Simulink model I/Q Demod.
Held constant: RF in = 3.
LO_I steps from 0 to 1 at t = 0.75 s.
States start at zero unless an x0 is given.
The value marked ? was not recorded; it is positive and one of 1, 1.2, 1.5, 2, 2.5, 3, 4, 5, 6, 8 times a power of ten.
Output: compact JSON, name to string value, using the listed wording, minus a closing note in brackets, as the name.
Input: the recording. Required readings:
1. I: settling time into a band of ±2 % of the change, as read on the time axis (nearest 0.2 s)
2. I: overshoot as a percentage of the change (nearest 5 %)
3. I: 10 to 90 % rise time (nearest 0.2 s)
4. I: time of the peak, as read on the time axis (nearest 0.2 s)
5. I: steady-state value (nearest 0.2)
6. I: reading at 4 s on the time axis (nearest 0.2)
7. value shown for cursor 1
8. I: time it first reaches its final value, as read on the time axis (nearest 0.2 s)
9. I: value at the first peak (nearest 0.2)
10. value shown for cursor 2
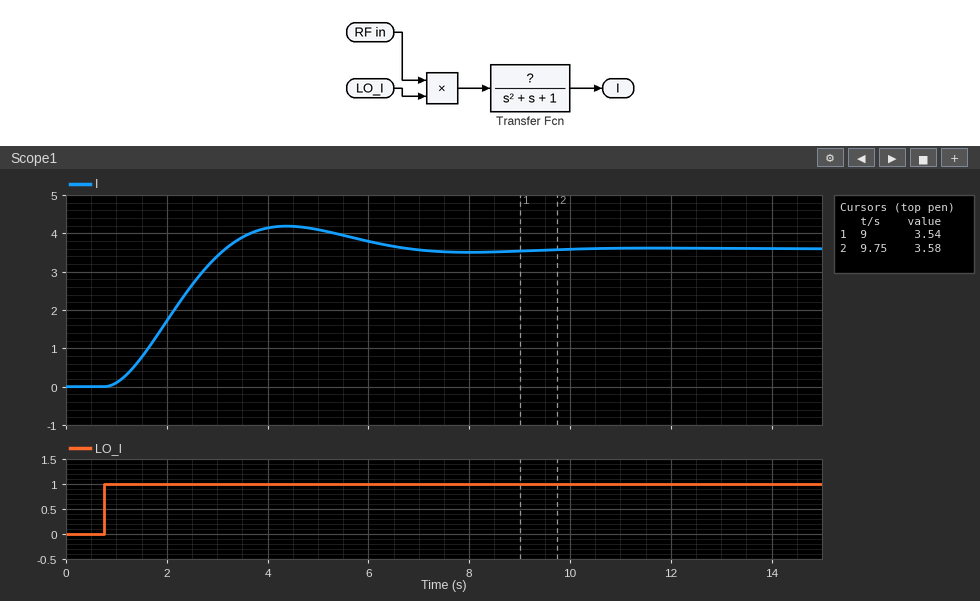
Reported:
{"I: settling time into a band of ±2 % of the change, as read on the time axis": "8.8 s", "I: overshoot as a percentage of the change": "15 %", "I: 10 to 90 % rise time": "1.6 s", "I: time of the peak, as read on the time axis": "4.4 s", "I: steady-state value": "3.6", "I: reading at 4 s on the time axis": "4.2", "value shown for cursor 1": "3.54", "I: time it first reaches its final value, as read on the time axis": "3.2 s", "I: value at the first peak": "4.2", "value shown for cursor 2": "3.58"}
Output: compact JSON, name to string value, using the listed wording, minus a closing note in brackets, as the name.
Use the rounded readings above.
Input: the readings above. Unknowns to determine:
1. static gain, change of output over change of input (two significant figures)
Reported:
{"static gain, change of output over change of input": "3.6"}
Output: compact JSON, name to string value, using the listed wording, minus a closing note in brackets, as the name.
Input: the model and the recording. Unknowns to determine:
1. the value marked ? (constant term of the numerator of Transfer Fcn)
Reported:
{"the value marked ?": "1.2"}
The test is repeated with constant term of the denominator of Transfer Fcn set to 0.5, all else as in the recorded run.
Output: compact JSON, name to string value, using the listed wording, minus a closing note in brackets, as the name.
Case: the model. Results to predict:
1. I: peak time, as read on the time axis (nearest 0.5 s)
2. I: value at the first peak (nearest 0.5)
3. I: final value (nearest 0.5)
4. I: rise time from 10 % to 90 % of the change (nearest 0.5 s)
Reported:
{"I: peak time, as read on the time axis": "7.0 s", "I: value at the first peak": "7.5", "I: final value": "7.0", "I: rise time from 10 % to 90 % of the change": "3.0 s"}
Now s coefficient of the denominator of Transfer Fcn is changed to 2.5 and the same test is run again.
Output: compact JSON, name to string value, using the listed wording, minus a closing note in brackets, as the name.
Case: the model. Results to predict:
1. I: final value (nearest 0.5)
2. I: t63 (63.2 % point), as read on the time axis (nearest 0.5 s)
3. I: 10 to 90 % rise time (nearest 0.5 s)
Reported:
{"I: final value": "3.5", "I: t63 (63.2 % point), as read on the time axis": "3.5 s", "I: 10 to 90 % rise time": "4.5 s"}
